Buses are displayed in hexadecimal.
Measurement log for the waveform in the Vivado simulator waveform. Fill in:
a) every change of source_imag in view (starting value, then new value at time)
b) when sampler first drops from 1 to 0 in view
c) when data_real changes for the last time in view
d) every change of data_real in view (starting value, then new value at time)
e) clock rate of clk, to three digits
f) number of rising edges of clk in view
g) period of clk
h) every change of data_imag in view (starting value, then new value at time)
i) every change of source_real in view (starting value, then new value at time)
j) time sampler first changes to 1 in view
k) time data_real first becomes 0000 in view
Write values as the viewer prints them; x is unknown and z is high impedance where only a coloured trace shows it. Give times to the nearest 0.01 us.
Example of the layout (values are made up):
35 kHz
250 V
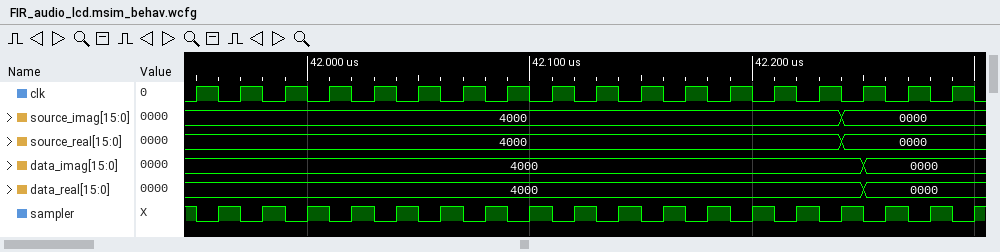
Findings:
4000, 0000 at 42.24 us
41.95 us
42.25 us
4000, 0000 at 42.25 us
50.0 MHz
18
0.02 us
4000, 0000 at 42.25 us
4000, 0000 at 42.24 us
41.96 us
42.25 us
